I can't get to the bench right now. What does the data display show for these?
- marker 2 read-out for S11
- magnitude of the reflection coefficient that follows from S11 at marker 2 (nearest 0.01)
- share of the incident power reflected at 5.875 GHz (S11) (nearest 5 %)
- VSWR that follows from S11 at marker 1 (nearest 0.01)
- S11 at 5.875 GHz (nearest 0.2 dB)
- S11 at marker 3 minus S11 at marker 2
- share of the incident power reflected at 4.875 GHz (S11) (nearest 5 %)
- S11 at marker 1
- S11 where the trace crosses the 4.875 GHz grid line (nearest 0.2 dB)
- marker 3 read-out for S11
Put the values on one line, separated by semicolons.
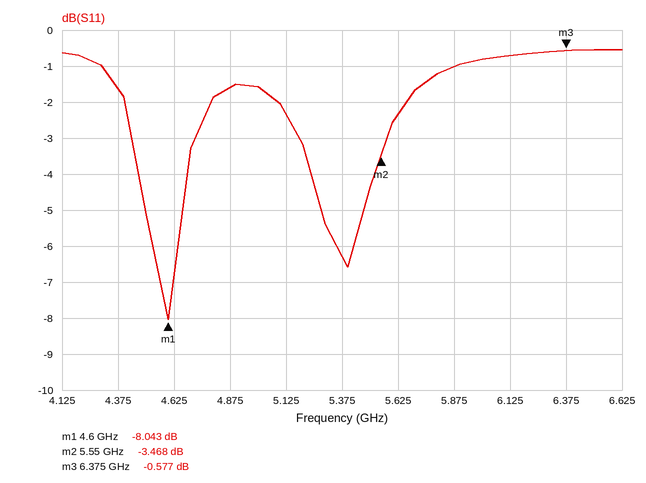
-3.468 dB; 0.67; 80 %; 2.31; -1.0 dB; 2.891 dB; 70 %; -8.043 dB; -1.6 dB; -0.577 dB
